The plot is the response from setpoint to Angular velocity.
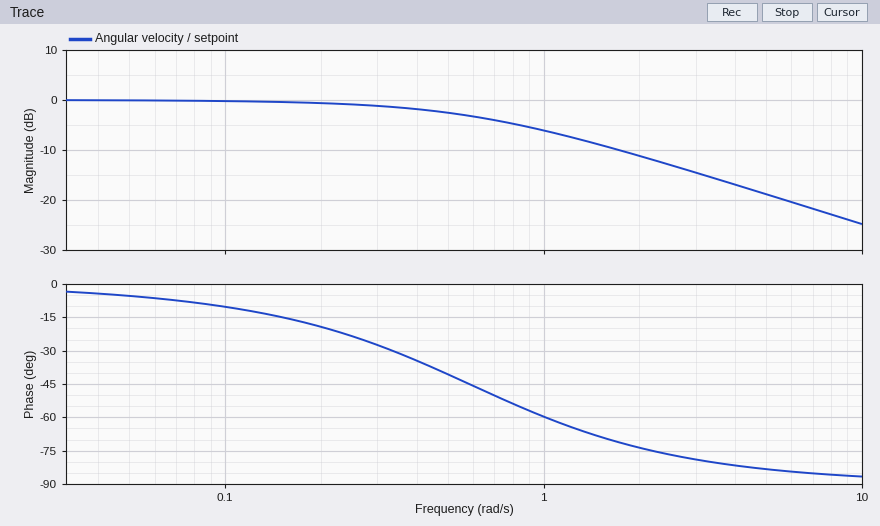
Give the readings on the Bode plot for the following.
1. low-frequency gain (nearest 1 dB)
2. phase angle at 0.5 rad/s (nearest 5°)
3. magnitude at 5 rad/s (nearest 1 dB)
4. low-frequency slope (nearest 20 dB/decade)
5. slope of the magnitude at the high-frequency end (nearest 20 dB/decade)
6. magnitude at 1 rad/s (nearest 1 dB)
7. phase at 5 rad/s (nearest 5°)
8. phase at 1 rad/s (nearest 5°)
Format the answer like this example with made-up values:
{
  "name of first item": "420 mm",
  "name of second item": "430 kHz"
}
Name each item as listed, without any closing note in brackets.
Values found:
{
  "low-frequency gain": "0 dB",
  "phase angle at 0.5 rad/s": "-40°",
  "magnitude at 5 rad/s": "-19 dB",
  "low-frequency slope": "0 dB/decade",
  "slope of the magnitude at the high-frequency end": "-20 dB/decade",
  "magnitude at 1 rad/s": "-6 dB",
  "phase at 5 rad/s": "-85°",
  "phase at 1 rad/s": "-60°"
}
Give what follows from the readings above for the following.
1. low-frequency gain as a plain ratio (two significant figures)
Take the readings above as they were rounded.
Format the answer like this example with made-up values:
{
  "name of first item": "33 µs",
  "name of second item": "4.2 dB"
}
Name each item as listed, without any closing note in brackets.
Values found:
{
  "low-frequency gain as a plain ratio": "1.0"
}
